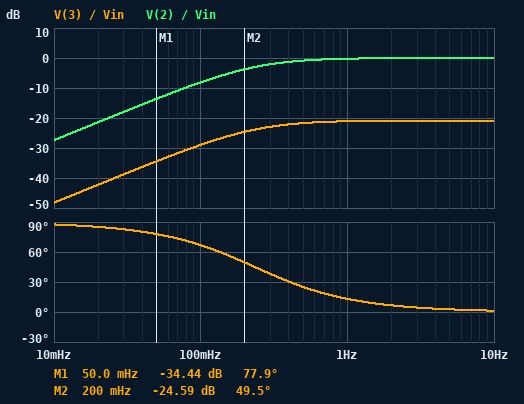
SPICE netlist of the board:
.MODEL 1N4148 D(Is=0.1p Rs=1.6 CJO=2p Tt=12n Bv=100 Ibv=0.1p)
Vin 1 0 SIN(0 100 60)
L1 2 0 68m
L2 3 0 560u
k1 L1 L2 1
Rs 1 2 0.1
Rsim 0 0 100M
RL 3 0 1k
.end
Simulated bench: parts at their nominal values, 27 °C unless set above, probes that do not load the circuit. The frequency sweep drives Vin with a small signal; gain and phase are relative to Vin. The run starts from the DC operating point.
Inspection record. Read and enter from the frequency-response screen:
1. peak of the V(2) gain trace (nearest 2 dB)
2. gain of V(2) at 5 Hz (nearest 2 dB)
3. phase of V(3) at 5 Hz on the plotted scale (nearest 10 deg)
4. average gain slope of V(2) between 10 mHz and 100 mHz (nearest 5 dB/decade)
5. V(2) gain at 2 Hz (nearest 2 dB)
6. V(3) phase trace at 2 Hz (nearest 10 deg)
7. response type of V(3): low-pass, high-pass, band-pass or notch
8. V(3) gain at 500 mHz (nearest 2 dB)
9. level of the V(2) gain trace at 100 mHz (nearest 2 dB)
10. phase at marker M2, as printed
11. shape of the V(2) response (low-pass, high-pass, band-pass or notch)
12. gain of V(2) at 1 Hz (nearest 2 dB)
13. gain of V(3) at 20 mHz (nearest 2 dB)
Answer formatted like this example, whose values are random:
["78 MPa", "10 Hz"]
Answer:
["0 dB", "0 dB", "0 deg", "20 dB/decade", "0 dB", "10 deg", "high-pass", "-22 dB", "-8 dB", "49.5 deg", "high-pass", "0 dB", "-42 dB"]
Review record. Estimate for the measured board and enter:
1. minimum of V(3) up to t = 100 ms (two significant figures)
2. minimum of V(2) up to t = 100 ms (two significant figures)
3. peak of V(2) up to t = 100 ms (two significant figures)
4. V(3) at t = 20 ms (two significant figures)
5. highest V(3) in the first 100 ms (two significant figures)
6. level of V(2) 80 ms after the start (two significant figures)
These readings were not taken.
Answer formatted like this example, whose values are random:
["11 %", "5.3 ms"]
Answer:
["-9.1 V", "-100 V", "100 V", "8.6 V", "9.0 V", "-95 V"]
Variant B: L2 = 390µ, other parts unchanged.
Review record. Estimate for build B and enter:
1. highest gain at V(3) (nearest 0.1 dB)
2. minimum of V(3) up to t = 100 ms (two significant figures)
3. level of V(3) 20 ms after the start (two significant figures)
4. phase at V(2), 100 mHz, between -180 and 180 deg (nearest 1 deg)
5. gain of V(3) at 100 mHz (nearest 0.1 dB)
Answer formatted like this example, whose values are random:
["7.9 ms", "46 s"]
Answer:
["-22.4 dB", "-7.6 V", "7.2 V", "67 deg", "-30.5 dB"]
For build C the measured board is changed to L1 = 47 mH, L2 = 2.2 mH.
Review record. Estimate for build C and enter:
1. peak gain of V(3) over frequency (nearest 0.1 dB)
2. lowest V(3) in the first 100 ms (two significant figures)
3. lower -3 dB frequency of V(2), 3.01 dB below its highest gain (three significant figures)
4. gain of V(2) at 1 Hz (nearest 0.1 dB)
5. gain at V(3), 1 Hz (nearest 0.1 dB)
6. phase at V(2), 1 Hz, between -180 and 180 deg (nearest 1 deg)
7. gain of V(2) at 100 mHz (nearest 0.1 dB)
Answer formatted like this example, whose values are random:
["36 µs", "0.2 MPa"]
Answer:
["-13.3 dB", "-22 V", "339 mHz", "-0.5 dB", "-13.8 dB", "19 deg", "-11.0 dB"]
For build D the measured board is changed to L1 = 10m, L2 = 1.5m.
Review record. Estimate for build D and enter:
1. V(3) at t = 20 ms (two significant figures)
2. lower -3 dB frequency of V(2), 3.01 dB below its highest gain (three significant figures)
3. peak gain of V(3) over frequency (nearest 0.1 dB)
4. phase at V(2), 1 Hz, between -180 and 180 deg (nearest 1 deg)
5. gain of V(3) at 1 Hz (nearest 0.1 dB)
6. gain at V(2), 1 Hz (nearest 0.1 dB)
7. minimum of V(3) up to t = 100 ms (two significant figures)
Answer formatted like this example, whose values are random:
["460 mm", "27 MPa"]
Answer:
["36 V", "1.59 Hz", "-8.2 dB", "58 deg", "-13.7 dB", "-5.5 dB", "-40 V"]
